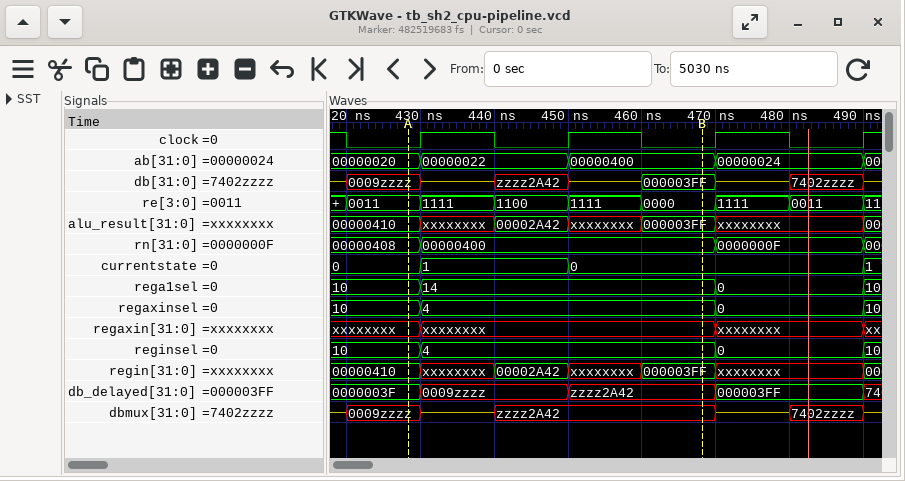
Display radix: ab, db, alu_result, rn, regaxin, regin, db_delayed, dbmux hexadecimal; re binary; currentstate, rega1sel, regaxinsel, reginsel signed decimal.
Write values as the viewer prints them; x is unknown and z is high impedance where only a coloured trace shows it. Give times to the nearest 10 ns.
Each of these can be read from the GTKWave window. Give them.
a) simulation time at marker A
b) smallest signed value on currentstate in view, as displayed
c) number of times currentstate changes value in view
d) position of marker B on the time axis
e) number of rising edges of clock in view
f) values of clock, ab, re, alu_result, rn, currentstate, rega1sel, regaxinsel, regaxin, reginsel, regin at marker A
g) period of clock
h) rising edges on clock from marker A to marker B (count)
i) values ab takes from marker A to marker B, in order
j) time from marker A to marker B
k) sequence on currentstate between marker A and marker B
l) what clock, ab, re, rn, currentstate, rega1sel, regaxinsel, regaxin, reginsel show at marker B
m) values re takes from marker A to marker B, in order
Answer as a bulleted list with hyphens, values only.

- 430 ns
- 0
- 3
- 470 ns
- 4
- clock=0, ab=00000020, re=0011, alu_result=00000410, rn=00000408, currentstate=0, rega1sel=10, regaxinsel=10, regaxin=xxxxxxxx, reginsel=10, regin=00000410
- 20 ns
- 2
- 00000020, 00000022, 00000400
- 40 ns
- 0, 1, 0
- clock=0, ab=00000400, re=0000, rn=00000400, currentstate=0, rega1sel=14, regaxinsel=4, regaxin=xxxxxxxx, reginsel=4
- 0011, 1111, 1100, 1111, 0000
